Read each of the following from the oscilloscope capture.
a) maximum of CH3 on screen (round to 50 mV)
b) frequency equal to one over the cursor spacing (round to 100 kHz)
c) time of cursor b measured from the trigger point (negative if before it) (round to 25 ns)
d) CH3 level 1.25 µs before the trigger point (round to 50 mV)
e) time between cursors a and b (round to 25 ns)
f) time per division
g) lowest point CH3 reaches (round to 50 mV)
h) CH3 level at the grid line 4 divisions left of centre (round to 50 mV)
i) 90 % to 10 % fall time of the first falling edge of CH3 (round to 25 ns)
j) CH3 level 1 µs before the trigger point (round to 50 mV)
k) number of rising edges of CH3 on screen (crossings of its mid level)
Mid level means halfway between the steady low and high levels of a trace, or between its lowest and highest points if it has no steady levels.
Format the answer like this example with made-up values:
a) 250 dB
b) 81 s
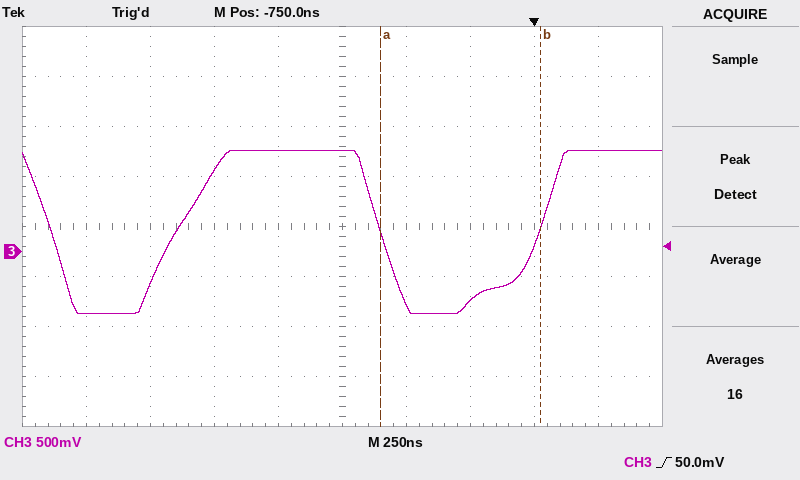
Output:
a) 1.00 V
b) 1.6 MHz
c) +25 ns
d) 800 mV
e) 625 ns
f) 250 ns
g) -600 mV
h) -600 mV
i) 175 ns
j) 1.00 V
k) 2
